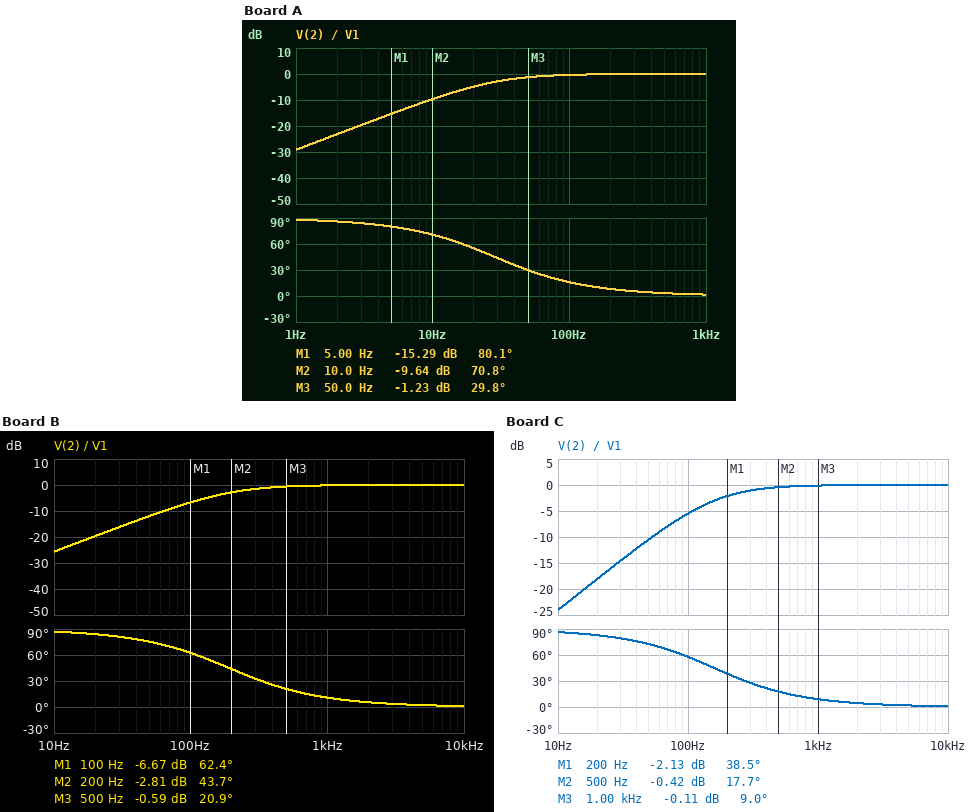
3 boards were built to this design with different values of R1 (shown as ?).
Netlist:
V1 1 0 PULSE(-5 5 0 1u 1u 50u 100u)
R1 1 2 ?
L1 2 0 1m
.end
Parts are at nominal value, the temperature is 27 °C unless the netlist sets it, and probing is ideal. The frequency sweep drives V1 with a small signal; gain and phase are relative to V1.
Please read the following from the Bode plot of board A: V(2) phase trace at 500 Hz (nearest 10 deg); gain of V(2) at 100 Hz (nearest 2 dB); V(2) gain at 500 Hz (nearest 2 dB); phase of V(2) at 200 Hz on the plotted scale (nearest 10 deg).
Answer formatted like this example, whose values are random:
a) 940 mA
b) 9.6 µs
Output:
a) 0 deg
b) 0 dB
c) 0 dB
d) 10 deg
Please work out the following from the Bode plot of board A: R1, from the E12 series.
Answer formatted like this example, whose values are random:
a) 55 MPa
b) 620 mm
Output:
a) 0.18 Ω
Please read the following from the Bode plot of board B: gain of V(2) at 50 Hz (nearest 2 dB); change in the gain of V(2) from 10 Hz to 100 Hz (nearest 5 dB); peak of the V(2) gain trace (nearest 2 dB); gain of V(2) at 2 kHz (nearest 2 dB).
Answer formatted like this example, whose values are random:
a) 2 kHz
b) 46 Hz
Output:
a) -12 dB
b) 20 dB
c) 0 dB
d) 0 dB
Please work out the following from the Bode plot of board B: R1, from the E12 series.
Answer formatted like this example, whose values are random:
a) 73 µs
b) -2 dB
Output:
a) 1.2 Ω
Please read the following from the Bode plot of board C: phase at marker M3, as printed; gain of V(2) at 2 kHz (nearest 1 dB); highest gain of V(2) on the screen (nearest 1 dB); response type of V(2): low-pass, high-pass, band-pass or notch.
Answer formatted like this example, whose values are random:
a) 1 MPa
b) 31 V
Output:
a) 9.0 deg
b) 0 dB
c) 0 dB
d) high-pass
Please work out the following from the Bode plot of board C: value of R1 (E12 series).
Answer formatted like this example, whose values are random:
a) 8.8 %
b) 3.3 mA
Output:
a) 1 Ω
